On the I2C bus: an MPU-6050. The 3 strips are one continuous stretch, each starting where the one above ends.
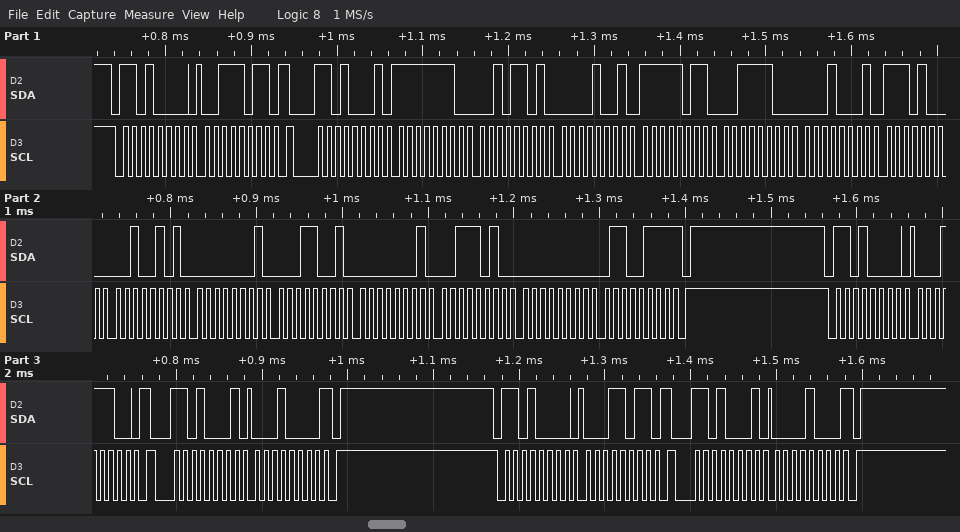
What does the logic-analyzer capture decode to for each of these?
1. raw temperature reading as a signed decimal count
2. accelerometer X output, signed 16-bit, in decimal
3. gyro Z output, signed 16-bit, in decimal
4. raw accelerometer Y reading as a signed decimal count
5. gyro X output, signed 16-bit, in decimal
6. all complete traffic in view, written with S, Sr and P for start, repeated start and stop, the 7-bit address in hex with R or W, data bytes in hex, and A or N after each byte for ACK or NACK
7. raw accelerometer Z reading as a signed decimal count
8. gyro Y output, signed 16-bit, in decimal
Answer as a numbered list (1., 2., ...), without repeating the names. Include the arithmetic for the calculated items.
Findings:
1. 0xE825 = -6107
2. 0xFE2D = -467
3. 0x0067 = 103
4. 0x09FB = 2555
5. 0x0119 = 281
6. S 68W A 3B A Sr 68R A FE A 2D A 09 A FB A 3C A 11 A E8 A 25 A 01 A 19 A 01 A 3A A 00 A 67 N P S 68W A 1C A Sr 68R A 10 N P S 68W A 1B A Sr 68R A 08 N P
7. 0x3C11 = 15377
8. 0x013A = 314
